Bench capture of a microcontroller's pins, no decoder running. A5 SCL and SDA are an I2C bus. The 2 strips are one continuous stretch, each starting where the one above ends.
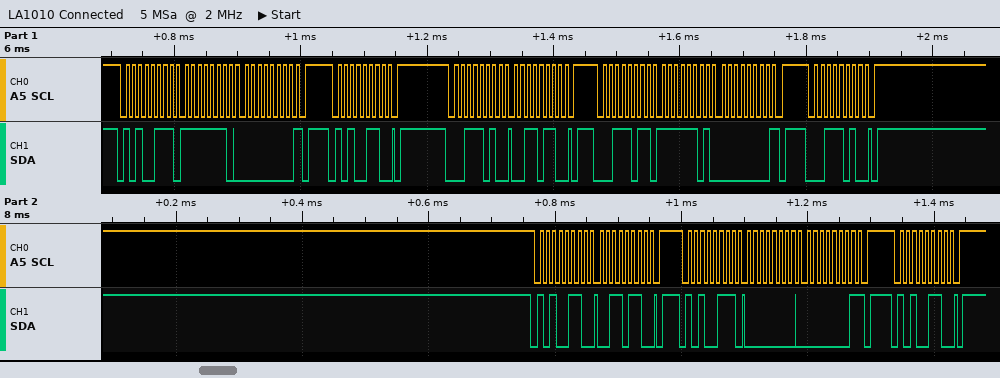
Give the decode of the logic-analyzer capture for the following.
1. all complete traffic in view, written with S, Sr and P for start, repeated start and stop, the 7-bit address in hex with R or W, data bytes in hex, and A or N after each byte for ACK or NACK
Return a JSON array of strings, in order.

["S 53R A FE A 00 N P S 53W A P S 1DW A 36 A P S 1DR A FD A 00 N P S 1DW A P S 53W A 36 A P S 53R A 00 A 01 N P S 53W A P"]
